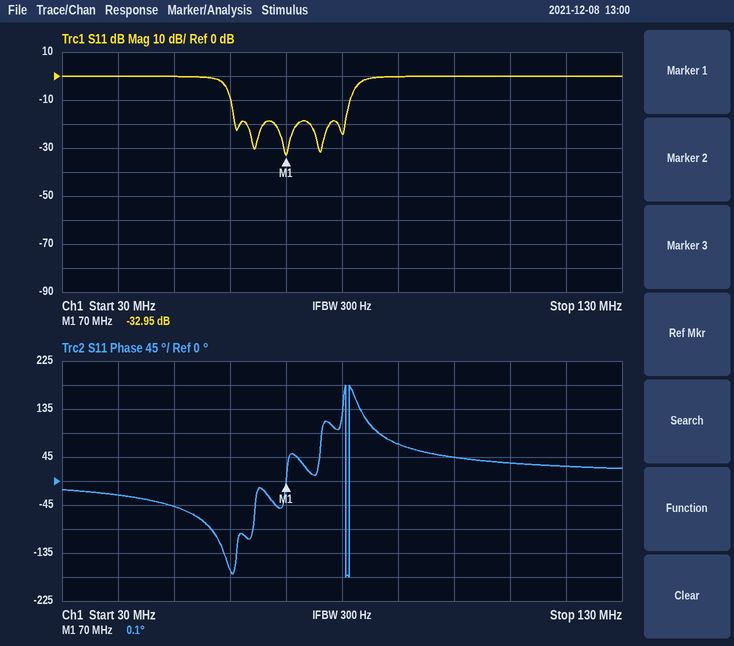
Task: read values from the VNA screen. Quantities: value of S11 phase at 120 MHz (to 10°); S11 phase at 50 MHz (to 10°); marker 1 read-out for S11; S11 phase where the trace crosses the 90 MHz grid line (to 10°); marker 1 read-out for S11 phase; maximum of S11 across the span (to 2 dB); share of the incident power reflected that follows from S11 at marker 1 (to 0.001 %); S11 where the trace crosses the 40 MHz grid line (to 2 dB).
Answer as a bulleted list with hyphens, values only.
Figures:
- 30°
- -50°
- -32.95 dB
- 70°
- 0.1°
- 0 dB
- 0.051 %
- 0 dB
